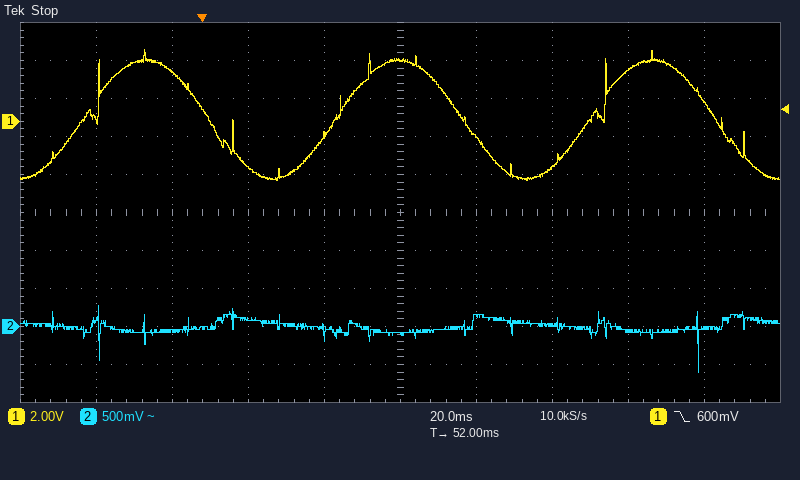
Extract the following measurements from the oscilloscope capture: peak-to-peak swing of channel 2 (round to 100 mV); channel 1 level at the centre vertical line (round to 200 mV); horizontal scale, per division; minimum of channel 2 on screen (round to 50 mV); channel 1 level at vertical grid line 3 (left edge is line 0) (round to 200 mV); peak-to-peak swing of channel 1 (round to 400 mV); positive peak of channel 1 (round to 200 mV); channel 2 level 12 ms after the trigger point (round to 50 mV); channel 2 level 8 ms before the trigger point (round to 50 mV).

900 mV
3.2 V
20 ms
-600 mV
-2.4 V
6.8 V
3.8 V
100 mV
-50 mV
